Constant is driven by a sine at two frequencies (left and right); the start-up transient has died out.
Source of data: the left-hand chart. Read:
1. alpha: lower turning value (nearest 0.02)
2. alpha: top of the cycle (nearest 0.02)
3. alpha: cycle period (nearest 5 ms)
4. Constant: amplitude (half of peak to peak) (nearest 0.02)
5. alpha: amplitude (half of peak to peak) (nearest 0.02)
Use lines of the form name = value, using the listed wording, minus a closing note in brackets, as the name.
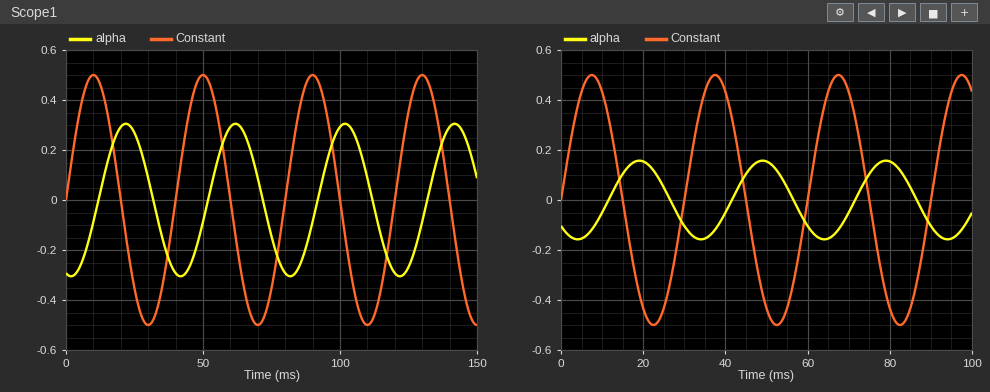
alpha: lower turning value = -0.30
alpha: top of the cycle = 0.30
alpha: cycle period = 40 ms
Constant: amplitude (half of peak to peak) = 0.50
alpha: amplitude (half of peak to peak) = 0.30
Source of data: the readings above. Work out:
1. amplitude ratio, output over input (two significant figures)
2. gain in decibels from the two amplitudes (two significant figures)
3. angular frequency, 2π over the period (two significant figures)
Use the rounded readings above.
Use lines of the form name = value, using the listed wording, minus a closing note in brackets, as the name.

amplitude ratio, output over input = 0.60
gain in decibels from the two amplitudes = -4.4 dB
angular frequency, 2π over the period = 0.16 rad/ms
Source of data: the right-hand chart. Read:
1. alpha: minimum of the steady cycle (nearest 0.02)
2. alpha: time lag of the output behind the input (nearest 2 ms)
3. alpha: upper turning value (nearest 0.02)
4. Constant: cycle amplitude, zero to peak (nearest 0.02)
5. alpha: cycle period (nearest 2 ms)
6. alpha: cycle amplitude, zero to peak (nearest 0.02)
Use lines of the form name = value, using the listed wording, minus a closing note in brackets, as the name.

alpha: minimum of the steady cycle = -0.16
alpha: time lag of the output behind the input = 12 ms
alpha: upper turning value = 0.16
Constant: cycle amplitude, zero to peak = 0.50
alpha: cycle period = 30 ms
alpha: cycle amplitude, zero to peak = 0.16
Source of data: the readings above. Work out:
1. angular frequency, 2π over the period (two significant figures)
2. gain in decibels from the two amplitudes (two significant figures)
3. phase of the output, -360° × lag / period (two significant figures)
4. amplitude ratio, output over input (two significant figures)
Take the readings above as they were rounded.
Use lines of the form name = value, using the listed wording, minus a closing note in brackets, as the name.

angular frequency, 2π over the period = 0.21 rad/ms
gain in decibels from the two amplitudes = -9.9 dB
phase of the output, -360° × lag / period = -140°
amplitude ratio, output over input = 0.32
